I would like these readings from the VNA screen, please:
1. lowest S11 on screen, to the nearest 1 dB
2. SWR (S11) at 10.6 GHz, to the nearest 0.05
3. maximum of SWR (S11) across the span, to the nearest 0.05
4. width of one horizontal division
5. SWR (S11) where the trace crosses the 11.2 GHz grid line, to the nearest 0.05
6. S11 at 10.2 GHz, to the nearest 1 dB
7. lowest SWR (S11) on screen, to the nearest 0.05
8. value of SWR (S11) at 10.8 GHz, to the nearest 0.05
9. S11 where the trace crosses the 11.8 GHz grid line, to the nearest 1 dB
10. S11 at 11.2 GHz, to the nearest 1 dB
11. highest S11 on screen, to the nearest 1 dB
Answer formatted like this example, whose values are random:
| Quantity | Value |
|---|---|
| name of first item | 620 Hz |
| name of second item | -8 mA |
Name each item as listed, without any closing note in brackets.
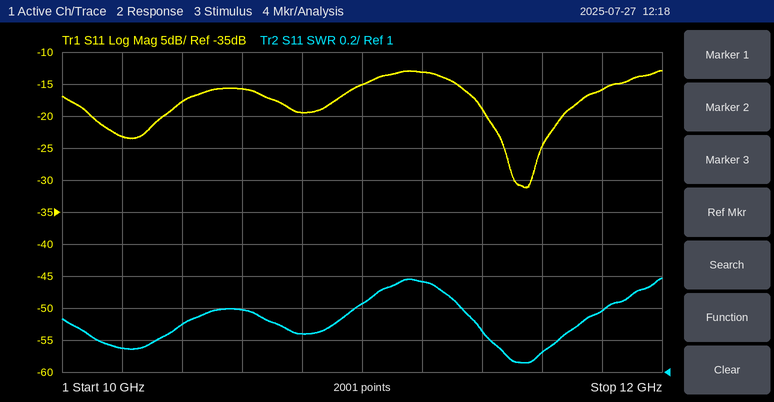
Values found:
| Quantity | Value |
|---|---|
| lowest S11 on screen, to the nearest 1 dB | -31 dB |
| SWR (S11) at 10.6 GHz, to the nearest 0.05 | 1.40 |
| maximum of SWR (S11) across the span, to the nearest 0.05 | 1.60 |
| width of one horizontal division | 200 MHz |
| SWR (S11) where the trace crosses the 11.2 GHz grid line, to the nearest 0.05 | 1.55 |
| S11 at 10.2 GHz, to the nearest 1 dB | -23 dB |
| lowest SWR (S11) on screen, to the nearest 0.05 | 1.05 |
| value of SWR (S11) at 10.8 GHz, to the nearest 0.05 | 1.25 |
| S11 where the trace crosses the 11.8 GHz grid line, to the nearest 1 dB | -16 dB |
| S11 at 11.2 GHz, to the nearest 1 dB | -13 dB |
| highest S11 on screen, to the nearest 1 dB | -13 dB |
